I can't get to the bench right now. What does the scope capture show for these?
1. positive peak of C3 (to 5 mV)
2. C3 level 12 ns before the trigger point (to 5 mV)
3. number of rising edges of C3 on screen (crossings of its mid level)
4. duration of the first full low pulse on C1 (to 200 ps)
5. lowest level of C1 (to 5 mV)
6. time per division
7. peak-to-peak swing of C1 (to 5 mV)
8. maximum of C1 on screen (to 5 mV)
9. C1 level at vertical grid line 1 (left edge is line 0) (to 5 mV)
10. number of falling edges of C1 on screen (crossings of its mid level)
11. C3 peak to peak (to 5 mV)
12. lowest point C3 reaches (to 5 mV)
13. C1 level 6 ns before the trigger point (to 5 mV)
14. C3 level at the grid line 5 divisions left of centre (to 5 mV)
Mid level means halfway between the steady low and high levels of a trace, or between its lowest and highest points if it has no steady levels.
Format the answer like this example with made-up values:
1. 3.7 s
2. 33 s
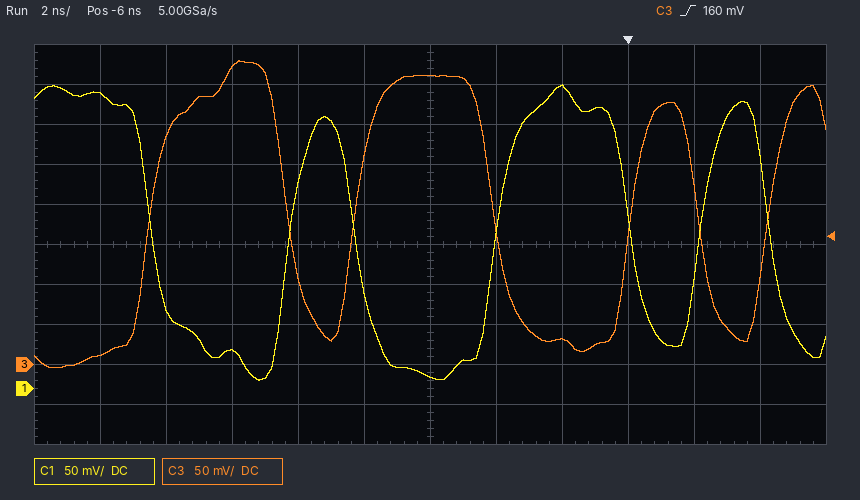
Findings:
1. 380 mV
2. 370 mV
3. 4
4. 4.2 ns
5. 10 mV
6. 2 ns
7. 370 mV
8. 380 mV
9. 370 mV
10. 4
11. 385 mV
12. -5 mV
13. 15 mV
14. 10 mV
